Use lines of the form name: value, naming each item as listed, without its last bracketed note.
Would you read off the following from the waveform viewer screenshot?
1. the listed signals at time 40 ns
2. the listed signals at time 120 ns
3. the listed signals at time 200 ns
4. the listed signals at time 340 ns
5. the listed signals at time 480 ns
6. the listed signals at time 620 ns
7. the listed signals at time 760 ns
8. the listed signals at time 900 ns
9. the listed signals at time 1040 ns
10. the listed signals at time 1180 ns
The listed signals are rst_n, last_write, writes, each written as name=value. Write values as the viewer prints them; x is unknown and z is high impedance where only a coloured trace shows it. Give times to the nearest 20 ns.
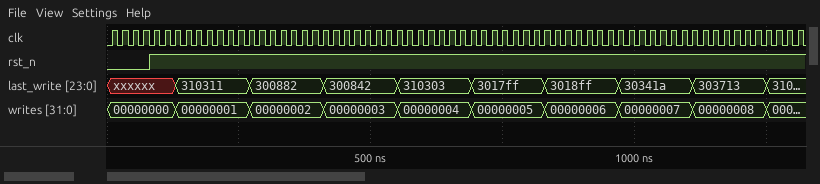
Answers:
the listed signals at time 40 ns: rst_n=0, last_write=xxxxxx, writes=00000000
the listed signals at time 120 ns: rst_n=1, last_write=xxxxxx, writes=00000000
the listed signals at time 200 ns: rst_n=1, last_write=310311, writes=00000001
the listed signals at time 340 ns: rst_n=1, last_write=300882, writes=00000002
the listed signals at time 480 ns: rst_n=1, last_write=300842, writes=00000003
the listed signals at time 620 ns: rst_n=1, last_write=310303, writes=00000004
the listed signals at time 760 ns: rst_n=1, last_write=3017ff, writes=00000005
the listed signals at time 900 ns: rst_n=1, last_write=3018ff, writes=00000006
the listed signals at time 1040 ns: rst_n=1, last_write=30341a, writes=00000007
the listed signals at time 1180 ns: rst_n=1, last_write=303713, writes=00000008
